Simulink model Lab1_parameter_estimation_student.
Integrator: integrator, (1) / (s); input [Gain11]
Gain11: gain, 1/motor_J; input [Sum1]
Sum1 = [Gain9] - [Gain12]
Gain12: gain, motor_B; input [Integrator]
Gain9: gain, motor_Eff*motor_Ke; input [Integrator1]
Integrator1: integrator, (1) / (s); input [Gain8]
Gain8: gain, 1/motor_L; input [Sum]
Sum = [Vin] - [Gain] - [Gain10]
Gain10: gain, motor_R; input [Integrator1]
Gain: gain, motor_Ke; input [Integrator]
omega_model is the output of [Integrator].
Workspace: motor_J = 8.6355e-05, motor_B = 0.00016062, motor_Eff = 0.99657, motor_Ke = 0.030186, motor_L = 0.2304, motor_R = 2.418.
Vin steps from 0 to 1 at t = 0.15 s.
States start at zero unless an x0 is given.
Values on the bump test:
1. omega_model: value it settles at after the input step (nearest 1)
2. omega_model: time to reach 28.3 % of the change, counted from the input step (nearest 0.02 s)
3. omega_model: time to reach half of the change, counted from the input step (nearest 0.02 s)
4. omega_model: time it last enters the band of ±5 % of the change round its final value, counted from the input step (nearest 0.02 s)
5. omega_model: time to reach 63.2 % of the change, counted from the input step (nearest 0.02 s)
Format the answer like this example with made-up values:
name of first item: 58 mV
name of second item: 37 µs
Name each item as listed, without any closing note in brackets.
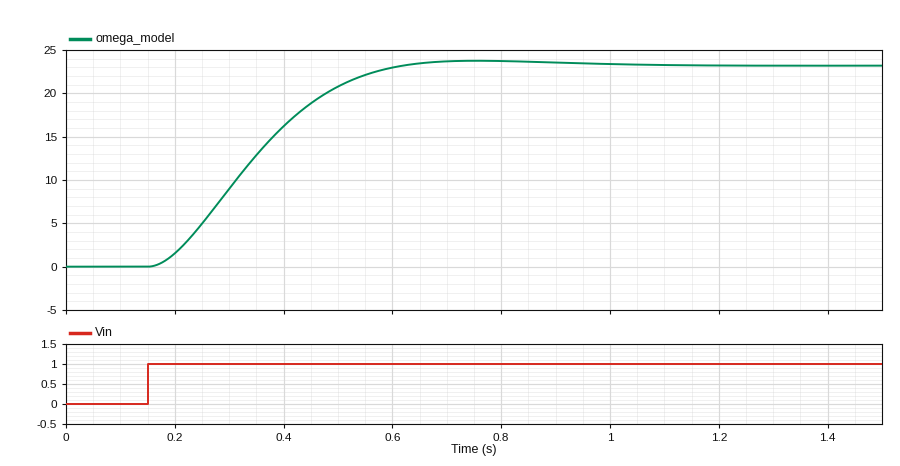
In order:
omega_model: value it settles at after the input step: 23
omega_model: time to reach 28.3 % of the change, counted from the input step: 0.12 s
omega_model: time to reach half of the change, counted from the input step: 0.18 s
omega_model: time it last enters the band of ±5 % of the change round its final value, counted from the input step: 0.40 s
omega_model: time to reach 63.2 % of the change, counted from the input step: 0.22 s
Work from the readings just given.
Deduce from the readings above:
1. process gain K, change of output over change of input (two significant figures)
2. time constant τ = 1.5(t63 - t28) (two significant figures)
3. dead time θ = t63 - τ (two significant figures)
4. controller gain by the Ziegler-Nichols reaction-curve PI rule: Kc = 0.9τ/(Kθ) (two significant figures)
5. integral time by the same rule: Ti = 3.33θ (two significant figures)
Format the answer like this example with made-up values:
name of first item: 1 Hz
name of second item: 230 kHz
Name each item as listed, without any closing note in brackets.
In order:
process gain K, change of output over change of input: 23
time constant τ = 1.5(t63 - t28): 0.15 s
dead time θ = t63 - τ: 0.070 s
controller gain by the Ziegler-Nichols reaction-curve PI rule: Kc = 0.9τ/(Kθ): 0.084
integral time by the same rule: Ti = 3.33θ: 0.23 s
